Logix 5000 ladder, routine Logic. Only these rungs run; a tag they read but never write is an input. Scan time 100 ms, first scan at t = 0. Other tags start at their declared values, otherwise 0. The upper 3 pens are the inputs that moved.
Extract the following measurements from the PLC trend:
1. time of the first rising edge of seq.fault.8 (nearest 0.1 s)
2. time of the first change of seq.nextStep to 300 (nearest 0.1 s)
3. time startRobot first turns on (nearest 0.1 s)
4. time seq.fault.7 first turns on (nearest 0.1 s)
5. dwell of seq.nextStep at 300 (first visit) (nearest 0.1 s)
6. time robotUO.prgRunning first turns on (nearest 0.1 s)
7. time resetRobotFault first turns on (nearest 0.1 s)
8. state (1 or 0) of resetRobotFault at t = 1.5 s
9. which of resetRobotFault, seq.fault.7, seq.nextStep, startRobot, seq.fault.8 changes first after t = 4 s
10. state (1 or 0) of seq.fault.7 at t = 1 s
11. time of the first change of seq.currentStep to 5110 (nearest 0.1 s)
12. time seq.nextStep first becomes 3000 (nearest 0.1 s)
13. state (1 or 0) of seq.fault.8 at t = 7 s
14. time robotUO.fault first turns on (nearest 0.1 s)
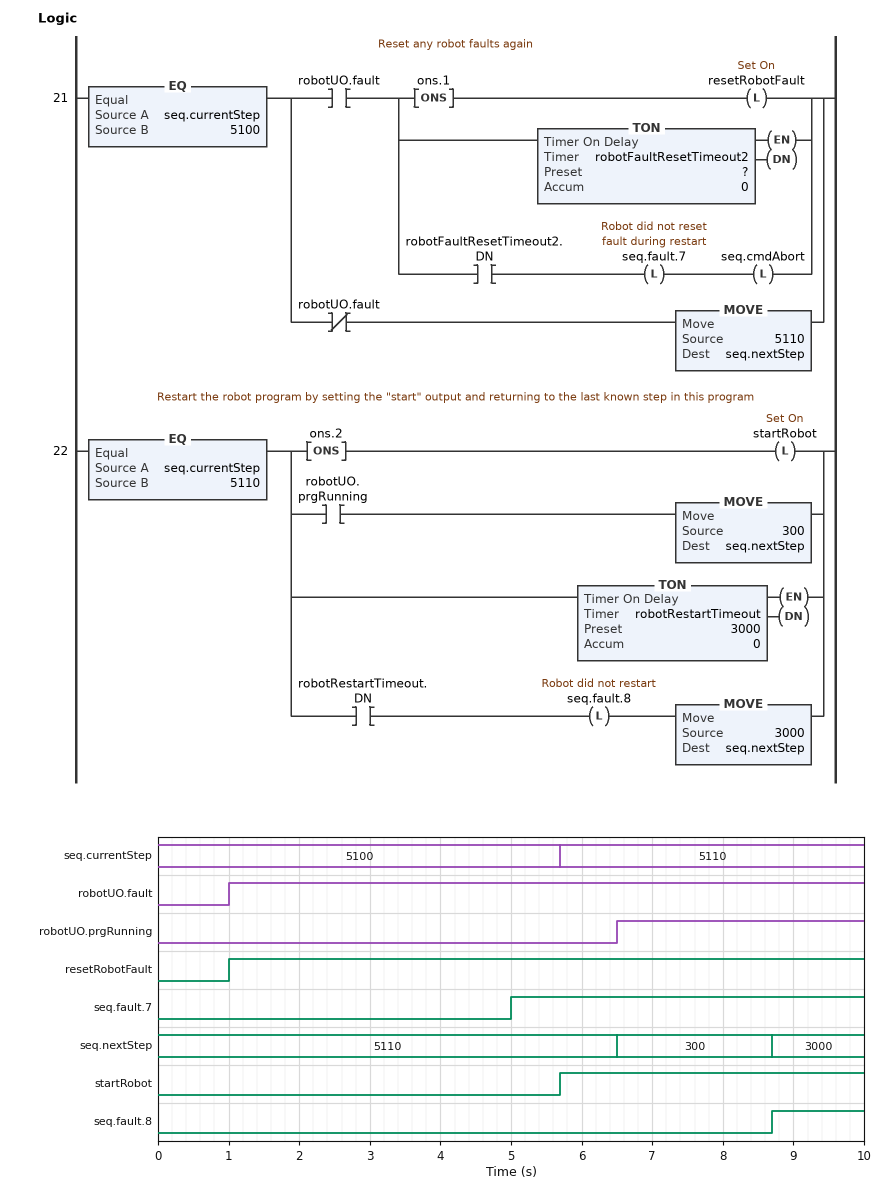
8.7 s
6.5 s
5.7 s
5.0 s
2.2 s
6.5 s
1.0 s
1
seq.fault.7
0
5.7 s
8.7 s
0
1.0 s
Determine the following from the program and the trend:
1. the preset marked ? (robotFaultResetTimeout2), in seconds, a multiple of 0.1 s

4.0 s
